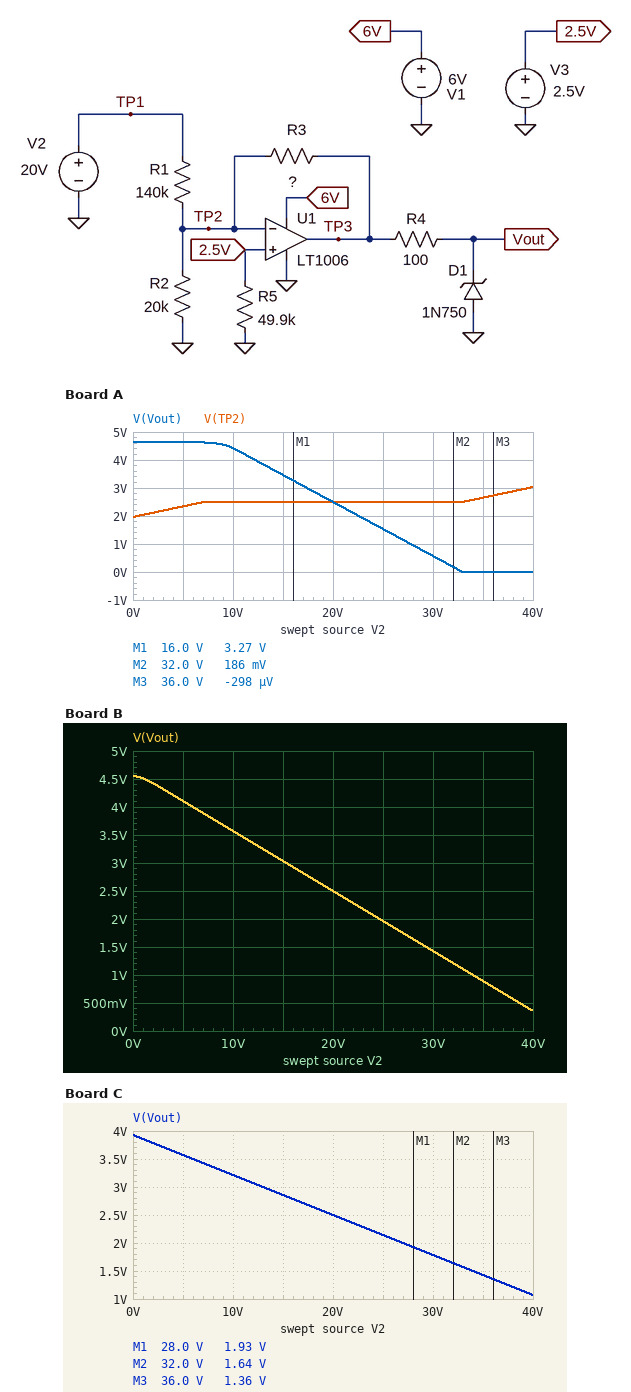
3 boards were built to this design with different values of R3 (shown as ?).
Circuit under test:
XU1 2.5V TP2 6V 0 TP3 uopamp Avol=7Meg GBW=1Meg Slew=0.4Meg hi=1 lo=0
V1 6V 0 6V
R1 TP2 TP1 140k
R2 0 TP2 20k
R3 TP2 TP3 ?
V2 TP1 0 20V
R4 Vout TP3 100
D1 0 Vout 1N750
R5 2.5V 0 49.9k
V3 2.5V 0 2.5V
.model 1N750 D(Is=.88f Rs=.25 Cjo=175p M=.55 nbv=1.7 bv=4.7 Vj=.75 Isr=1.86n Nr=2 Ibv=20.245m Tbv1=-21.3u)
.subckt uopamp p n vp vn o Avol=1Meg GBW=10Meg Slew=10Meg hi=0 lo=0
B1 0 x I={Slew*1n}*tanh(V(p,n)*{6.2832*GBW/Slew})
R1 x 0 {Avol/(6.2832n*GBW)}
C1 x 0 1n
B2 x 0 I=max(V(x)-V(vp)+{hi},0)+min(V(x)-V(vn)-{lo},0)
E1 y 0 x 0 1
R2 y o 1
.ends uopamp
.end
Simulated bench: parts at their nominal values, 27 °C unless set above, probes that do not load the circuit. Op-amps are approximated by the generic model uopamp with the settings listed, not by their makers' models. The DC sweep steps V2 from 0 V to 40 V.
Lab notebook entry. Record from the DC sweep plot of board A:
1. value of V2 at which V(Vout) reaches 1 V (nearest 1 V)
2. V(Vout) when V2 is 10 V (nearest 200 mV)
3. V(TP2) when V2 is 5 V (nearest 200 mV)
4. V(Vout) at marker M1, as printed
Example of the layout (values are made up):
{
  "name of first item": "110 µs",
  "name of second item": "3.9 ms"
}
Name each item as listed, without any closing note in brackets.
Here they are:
{
  "value of V2 at which V(Vout) reaches 1 V": "28 V",
  "V(Vout) when V2 is 10 V": "4.4 V",
  "V(TP2) when V2 is 5 V": "2.4 V",
  "V(Vout) at marker M1, as printed": "3.27 V"
}
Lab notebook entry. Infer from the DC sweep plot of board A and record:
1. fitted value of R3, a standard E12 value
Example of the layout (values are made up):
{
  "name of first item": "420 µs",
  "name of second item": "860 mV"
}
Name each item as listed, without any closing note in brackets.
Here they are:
{
  "fitted value of R3, a standard E12 value": "27 kΩ"
}
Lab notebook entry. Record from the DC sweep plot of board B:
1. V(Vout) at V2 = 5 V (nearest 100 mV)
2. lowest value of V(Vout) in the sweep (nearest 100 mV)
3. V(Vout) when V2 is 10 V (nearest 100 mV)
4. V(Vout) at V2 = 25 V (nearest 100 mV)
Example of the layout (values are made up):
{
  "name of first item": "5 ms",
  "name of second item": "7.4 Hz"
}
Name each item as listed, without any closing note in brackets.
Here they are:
{
  "V(Vout) at V2 = 5 V": "4.1 V",
  "lowest value of V(Vout) in the sweep": "400 mV",
  "V(Vout) when V2 is 10 V": "3.6 V",
  "V(Vout) at V2 = 25 V": "2.0 V"
}
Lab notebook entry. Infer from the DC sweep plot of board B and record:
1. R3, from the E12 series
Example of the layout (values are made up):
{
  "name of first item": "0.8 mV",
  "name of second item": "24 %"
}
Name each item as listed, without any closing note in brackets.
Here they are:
{
  "R3, from the E12 series": "15 kΩ"
}
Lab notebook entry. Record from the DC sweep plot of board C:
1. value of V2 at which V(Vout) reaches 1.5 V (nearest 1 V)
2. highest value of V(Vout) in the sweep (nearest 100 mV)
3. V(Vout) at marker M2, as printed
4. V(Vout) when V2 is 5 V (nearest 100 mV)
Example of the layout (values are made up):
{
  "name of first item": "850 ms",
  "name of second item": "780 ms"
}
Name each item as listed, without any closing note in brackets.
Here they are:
{
  "value of V2 at which V(Vout) reaches 1.5 V": "34 V",
  "highest value of V(Vout) in the sweep": "3.9 V",
  "V(Vout) at marker M2, as printed": "1.64 V",
  "V(Vout) when V2 is 5 V": "3.6 V"
}
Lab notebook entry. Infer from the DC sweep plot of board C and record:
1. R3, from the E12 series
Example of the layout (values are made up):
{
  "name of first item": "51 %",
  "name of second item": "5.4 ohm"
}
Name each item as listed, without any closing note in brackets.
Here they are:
{
  "R3, from the E12 series": "10 kΩ"
}
